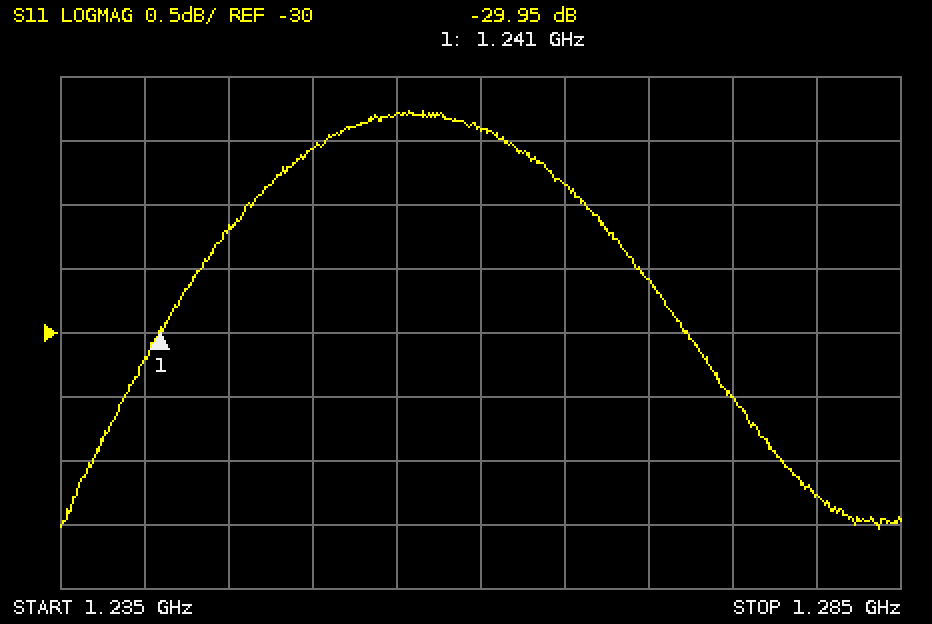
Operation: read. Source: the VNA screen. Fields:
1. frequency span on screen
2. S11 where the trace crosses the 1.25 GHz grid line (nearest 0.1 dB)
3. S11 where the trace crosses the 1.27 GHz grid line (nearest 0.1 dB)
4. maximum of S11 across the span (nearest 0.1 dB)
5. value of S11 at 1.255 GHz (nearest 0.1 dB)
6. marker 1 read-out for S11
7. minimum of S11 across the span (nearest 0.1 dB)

50 MHz
-28.6 dB
-29.6 dB
-28.3 dB
-28.3 dB
-29.95 dB
-31.5 dB
